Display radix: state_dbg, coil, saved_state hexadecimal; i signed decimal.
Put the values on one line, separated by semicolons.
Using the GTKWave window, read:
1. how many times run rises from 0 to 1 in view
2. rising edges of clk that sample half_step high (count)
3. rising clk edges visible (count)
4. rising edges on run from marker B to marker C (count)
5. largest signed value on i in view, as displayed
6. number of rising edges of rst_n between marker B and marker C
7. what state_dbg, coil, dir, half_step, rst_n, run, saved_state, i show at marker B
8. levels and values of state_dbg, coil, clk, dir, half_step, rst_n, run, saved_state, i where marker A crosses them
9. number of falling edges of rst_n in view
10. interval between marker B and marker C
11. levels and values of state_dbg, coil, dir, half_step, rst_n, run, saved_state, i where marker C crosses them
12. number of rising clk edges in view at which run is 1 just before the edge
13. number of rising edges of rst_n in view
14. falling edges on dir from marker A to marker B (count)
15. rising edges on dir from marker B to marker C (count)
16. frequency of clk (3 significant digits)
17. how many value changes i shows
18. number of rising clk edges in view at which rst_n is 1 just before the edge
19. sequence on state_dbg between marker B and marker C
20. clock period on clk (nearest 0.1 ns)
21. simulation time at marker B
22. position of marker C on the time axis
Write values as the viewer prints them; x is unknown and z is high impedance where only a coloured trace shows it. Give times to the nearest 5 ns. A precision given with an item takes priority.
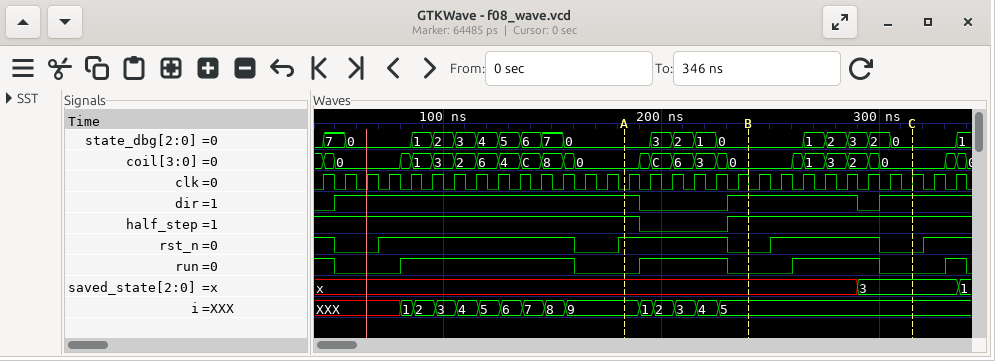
4; 26; 30; 1; 9; 1; state_dbg=0, coil=0, dir=1, half_step=1, rst_n=0, run=0, saved_state=x, i=5; state_dbg=0, coil=0, clk=0, dir=1, half_step=1, rst_n=1, run=0, saved_state=x, i=9; 4; 75 ns; state_dbg=0, coil=0, dir=1, half_step=1, rst_n=0, run=0, saved_state=3, i=5; 18; 4; 1; 1; 100 MHz; 14; 22; 0, 1, 2, 3, 2, 0; 10 ns; 240 ns; 315 ns
